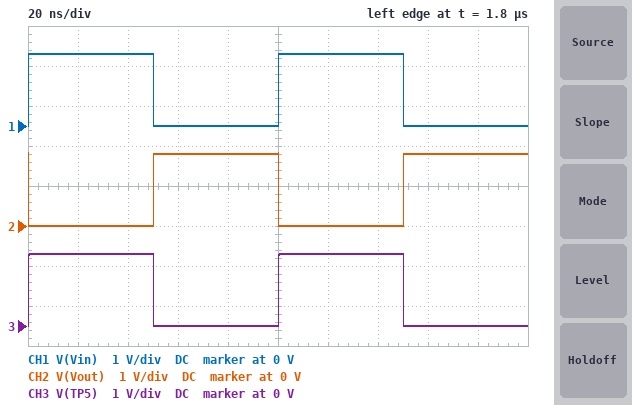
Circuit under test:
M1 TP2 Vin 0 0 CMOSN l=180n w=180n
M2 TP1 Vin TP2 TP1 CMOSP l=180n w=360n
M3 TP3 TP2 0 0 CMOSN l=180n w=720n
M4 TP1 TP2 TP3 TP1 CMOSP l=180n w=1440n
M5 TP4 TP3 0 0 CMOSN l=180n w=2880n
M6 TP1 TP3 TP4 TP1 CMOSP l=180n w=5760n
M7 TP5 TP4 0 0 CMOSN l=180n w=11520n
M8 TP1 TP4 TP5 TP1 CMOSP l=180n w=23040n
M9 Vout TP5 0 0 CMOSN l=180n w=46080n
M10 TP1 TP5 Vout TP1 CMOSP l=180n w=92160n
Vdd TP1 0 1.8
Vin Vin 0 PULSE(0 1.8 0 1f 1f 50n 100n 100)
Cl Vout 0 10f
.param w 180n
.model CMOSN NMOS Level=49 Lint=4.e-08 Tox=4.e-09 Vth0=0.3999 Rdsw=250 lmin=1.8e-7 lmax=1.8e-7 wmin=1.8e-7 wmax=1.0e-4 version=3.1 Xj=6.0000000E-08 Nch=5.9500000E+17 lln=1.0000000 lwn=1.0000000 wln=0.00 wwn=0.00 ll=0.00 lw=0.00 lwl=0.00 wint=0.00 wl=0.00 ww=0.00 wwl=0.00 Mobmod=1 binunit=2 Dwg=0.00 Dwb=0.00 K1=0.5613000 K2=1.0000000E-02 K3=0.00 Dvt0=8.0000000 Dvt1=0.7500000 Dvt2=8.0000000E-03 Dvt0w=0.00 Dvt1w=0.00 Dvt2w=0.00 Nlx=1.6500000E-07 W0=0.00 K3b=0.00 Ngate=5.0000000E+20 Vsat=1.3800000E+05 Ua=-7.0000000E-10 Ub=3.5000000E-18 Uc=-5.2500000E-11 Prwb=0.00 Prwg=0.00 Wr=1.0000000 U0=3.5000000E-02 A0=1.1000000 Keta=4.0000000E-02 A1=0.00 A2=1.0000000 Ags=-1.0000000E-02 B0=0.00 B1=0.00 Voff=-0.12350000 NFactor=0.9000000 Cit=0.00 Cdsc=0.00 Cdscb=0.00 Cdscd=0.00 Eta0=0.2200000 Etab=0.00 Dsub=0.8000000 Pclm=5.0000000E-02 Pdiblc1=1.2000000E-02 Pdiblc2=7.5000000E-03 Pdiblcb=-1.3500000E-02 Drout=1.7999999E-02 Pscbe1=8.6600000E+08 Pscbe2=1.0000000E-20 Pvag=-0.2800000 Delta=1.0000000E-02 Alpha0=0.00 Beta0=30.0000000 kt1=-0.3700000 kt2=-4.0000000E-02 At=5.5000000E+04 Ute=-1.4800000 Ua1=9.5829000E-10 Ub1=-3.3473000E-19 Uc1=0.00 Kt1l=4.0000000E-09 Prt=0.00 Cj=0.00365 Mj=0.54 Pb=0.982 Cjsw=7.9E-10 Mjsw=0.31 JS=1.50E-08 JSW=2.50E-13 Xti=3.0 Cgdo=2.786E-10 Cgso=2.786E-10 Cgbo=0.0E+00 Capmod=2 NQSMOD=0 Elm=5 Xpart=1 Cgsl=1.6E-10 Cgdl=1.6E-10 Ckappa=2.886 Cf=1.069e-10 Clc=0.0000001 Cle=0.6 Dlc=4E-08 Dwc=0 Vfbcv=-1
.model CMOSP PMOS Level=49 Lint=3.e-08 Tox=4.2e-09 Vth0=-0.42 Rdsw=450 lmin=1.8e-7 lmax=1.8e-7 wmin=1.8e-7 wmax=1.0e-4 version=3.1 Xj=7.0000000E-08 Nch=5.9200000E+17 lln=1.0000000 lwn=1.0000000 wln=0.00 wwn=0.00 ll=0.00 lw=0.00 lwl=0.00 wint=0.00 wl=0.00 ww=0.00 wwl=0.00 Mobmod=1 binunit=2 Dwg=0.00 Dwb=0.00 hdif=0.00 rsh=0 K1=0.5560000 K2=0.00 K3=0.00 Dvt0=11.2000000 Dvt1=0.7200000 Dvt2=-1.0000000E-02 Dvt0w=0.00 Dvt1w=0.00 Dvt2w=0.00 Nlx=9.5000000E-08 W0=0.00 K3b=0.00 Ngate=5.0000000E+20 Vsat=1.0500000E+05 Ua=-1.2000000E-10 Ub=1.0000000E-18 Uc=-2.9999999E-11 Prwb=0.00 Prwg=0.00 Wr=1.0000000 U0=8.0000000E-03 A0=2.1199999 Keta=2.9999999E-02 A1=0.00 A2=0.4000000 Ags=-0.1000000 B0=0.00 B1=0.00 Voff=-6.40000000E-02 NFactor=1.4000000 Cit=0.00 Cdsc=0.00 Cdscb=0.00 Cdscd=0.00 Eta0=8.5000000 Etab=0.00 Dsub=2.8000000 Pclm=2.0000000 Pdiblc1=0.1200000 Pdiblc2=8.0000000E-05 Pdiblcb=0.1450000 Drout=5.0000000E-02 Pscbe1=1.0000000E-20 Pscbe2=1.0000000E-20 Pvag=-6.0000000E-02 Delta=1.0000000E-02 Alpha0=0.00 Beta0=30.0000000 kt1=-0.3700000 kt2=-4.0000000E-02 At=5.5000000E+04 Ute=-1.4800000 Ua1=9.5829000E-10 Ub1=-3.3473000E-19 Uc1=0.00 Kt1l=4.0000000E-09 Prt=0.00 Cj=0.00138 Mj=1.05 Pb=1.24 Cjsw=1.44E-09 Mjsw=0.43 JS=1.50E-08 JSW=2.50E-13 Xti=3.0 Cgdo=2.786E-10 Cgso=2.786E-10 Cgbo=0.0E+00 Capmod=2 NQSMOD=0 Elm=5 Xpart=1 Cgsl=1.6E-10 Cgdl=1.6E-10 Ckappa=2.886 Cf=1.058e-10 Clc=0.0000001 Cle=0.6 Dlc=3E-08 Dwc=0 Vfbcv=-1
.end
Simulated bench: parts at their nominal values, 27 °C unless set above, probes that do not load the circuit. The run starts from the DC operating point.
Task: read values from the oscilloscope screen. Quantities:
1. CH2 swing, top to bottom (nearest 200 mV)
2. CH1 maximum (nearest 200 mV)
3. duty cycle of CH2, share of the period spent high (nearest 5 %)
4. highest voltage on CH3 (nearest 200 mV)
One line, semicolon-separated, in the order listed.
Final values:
1.8 V; 1.8 V; 50 %; 1.8 V
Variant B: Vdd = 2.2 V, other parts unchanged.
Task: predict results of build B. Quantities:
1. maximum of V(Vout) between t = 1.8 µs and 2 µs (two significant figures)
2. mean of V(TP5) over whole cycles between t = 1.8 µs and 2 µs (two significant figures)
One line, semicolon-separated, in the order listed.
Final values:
2.2 V; 1.1 V
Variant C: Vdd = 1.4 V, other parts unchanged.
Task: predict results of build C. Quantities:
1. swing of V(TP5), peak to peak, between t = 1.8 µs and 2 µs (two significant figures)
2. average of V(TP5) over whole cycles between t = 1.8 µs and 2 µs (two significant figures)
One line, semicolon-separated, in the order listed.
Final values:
1.4 V; 700 mV
